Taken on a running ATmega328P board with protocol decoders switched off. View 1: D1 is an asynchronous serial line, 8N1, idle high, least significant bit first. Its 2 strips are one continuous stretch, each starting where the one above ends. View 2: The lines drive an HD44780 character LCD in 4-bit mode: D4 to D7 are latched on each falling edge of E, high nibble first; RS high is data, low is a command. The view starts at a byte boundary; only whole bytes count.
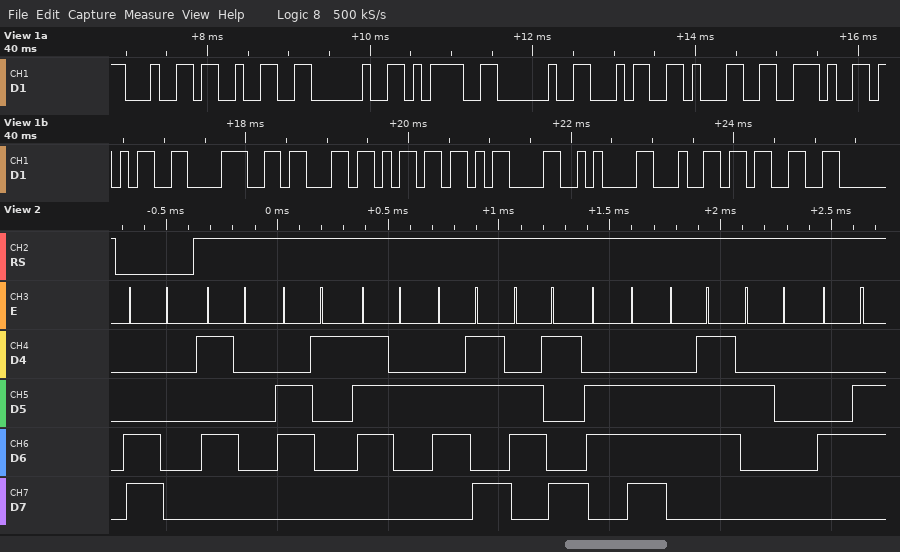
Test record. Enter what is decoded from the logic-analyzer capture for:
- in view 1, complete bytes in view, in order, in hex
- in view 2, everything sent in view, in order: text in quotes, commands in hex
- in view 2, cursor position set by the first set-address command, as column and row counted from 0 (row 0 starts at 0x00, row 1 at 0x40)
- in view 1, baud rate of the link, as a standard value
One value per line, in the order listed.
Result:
64 32 20 3D 20 34 31 2E 35 38 63 6D 0D 0A 64 33
0xC0 "Parking F"
column 0, row 1
9600 baud
